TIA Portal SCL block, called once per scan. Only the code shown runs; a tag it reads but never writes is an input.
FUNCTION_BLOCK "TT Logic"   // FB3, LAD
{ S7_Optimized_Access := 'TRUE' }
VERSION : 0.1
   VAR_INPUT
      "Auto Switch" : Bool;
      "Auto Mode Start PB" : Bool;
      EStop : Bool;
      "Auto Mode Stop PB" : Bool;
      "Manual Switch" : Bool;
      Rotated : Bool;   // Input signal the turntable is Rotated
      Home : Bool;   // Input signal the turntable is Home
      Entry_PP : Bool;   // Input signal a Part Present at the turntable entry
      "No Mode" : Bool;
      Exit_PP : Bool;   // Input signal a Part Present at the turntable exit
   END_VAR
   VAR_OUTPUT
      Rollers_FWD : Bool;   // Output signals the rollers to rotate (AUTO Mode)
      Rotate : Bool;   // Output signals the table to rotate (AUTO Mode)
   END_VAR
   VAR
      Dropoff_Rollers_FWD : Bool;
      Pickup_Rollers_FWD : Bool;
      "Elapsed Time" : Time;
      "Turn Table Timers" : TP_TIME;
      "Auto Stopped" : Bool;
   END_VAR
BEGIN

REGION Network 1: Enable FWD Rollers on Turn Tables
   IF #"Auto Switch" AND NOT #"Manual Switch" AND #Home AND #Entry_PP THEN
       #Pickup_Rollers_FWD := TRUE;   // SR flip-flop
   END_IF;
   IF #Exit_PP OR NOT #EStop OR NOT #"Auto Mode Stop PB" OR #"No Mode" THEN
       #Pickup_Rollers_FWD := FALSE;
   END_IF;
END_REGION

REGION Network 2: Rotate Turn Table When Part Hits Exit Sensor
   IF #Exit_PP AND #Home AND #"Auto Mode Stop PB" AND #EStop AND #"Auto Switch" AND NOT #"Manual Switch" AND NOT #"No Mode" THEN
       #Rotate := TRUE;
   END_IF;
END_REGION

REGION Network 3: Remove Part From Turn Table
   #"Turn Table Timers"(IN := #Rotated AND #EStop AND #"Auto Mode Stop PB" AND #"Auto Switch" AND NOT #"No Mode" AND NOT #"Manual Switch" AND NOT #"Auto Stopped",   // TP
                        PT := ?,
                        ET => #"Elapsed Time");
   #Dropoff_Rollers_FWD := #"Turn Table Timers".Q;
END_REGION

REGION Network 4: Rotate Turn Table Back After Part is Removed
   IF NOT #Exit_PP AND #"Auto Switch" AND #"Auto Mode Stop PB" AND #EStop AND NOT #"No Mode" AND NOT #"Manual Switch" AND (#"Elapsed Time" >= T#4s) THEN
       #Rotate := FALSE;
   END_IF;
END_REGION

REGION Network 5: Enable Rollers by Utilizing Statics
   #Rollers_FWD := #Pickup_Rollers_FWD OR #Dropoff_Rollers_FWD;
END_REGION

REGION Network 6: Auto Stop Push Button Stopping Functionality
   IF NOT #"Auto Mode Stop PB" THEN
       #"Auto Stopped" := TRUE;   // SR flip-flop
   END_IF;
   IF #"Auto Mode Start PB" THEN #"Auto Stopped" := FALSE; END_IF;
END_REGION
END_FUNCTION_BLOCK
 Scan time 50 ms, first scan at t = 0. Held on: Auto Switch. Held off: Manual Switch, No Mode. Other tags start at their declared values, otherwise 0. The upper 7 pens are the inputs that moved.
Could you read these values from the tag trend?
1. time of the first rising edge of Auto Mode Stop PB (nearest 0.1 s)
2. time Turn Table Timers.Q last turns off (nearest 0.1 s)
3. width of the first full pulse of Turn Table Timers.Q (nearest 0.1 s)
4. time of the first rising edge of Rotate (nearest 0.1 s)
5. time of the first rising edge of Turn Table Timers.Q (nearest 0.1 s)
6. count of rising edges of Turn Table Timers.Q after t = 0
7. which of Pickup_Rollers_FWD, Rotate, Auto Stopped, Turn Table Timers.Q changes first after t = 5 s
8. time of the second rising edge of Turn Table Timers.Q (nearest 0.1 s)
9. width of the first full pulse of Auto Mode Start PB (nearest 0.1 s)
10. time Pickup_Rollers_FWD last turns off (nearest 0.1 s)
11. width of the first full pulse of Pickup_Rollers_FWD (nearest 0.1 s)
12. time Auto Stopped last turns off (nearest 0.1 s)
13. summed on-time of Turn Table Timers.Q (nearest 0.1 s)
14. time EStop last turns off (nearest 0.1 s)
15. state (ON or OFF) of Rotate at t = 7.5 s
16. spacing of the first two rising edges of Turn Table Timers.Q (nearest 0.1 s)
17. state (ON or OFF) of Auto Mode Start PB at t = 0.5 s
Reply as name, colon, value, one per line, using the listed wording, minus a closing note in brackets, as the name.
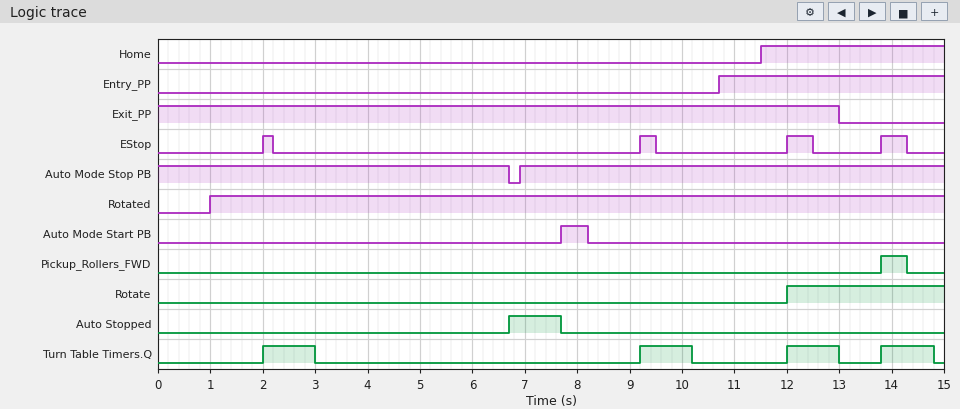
time of the first rising edge of Auto Mode Stop PB: 6.9 s
time Turn Table Timers.Q last turns off: 14.8 s
width of the first full pulse of Turn Table Timers.Q: 1.0 s
time of the first rising edge of Rotate: 12.0 s
time of the first rising edge of Turn Table Timers.Q: 2.0 s
count of rising edges of Turn Table Timers.Q after t = 0: 4
which of Pickup_Rollers_FWD, Rotate, Auto Stopped, Turn Table Timers.Q changes first after t = 5 s: Auto Stopped
time of the second rising edge of Turn Table Timers.Q: 9.2 s
width of the first full pulse of Auto Mode Start PB: 0.5 s
time Pickup_Rollers_FWD last turns off: 14.3 s
width of the first full pulse of Pickup_Rollers_FWD: 0.5 s
time Auto Stopped last turns off: 7.7 s
summed on-time of Turn Table Timers.Q: 4.0 s
time EStop last turns off: 14.3 s
state (ON or OFF) of Rotate at t = 7.5 s: OFF
spacing of the first two rising edges of Turn Table Timers.Q: 7.2 s
state (ON or OFF) of Auto Mode Start PB at t = 0.5 s: OFF
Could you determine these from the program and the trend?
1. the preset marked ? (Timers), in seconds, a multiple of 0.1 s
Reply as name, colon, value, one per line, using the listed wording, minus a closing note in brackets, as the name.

the preset marked ? (Timers), in seconds, a multiple of 0.1 s: 1.0 s
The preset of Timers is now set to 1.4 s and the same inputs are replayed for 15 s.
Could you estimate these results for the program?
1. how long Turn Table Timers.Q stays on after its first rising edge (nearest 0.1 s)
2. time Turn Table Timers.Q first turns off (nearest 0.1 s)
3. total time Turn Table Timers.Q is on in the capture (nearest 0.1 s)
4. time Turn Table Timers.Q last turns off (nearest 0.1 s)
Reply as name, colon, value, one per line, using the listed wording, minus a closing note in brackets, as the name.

how long Turn Table Timers.Q stays on after its first rising edge: 1.4 s
time Turn Table Timers.Q first turns off: 3.4 s
total time Turn Table Timers.Q is on in the capture: 5.4 s
time Turn Table Timers.Q last turns off: 13.4 s
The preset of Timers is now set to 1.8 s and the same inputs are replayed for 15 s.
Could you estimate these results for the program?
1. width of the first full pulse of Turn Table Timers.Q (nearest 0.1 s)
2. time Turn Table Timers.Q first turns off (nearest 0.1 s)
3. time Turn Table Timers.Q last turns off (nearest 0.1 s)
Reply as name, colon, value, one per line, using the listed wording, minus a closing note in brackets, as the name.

width of the first full pulse of Turn Table Timers.Q: 1.8 s
time Turn Table Timers.Q first turns off: 3.8 s
time Turn Table Timers.Q last turns off: 13.8 s
